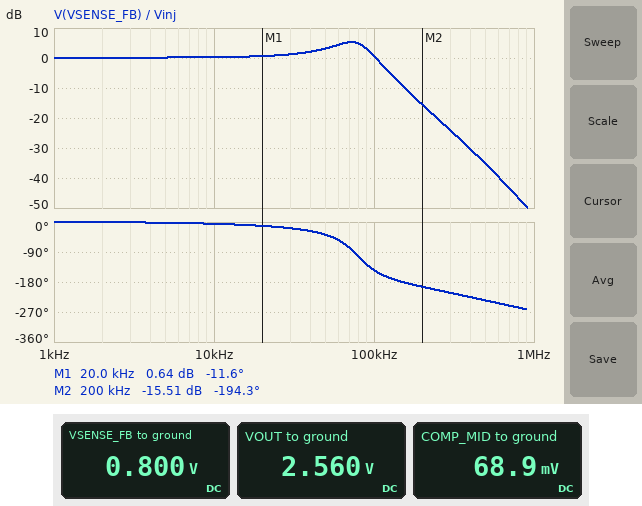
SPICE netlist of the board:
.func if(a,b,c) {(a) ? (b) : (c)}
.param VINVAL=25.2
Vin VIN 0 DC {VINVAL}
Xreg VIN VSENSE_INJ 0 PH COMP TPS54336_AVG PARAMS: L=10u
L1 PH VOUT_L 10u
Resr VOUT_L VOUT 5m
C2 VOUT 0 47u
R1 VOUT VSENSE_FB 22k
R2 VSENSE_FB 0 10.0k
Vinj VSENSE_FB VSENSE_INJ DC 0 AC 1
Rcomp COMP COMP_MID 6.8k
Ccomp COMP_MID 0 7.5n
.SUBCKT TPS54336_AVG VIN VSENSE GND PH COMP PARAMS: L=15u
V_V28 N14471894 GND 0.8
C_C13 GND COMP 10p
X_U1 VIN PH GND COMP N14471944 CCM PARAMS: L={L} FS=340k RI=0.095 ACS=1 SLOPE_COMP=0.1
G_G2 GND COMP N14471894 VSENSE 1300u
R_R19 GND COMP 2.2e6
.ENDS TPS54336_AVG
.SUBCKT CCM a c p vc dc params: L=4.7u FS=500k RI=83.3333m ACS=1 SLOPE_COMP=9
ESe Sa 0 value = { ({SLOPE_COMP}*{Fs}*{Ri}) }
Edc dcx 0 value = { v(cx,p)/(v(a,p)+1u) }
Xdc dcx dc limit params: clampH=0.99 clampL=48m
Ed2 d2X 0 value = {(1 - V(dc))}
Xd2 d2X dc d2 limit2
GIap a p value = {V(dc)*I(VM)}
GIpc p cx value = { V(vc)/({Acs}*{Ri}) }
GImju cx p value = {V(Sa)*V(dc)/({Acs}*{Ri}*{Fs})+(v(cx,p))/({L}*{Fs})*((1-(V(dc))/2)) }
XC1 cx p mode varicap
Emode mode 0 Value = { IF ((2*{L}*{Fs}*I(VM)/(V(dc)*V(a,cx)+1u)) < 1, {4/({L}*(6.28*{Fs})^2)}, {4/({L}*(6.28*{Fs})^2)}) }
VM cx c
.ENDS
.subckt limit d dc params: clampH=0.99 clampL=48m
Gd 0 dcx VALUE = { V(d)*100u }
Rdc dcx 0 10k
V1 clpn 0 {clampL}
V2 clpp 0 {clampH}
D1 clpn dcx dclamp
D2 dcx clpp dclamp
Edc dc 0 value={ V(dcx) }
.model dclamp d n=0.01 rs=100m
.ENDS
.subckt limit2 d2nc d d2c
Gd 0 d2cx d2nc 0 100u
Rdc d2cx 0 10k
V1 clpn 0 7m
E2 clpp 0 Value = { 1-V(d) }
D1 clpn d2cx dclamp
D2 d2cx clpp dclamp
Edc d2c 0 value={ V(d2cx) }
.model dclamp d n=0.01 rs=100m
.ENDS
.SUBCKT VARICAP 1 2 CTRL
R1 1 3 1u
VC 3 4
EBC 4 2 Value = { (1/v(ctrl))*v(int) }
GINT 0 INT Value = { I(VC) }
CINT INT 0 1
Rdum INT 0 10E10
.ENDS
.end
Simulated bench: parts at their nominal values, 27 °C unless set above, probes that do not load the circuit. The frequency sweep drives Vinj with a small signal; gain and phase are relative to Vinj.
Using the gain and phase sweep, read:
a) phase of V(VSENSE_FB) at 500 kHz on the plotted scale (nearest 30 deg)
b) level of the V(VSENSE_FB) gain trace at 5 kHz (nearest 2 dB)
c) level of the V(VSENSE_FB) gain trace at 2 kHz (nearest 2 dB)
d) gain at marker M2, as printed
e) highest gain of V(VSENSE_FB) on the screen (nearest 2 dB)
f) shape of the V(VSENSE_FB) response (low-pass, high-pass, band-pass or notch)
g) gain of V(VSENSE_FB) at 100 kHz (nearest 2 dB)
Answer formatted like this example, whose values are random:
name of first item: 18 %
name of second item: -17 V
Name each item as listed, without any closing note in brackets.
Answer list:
phase of V(VSENSE_FB) at 500 kHz on the plotted scale: -240 deg
level of the V(VSENSE_FB) gain trace at 5 kHz: 0 dB
level of the V(VSENSE_FB) gain trace at 2 kHz: 0 dB
gain at marker M2, as printed: -15.51 dB
highest gain of V(VSENSE_FB) on the screen: 6 dB
shape of the V(VSENSE_FB) response: low-pass
gain of V(VSENSE_FB) at 100 kHz: 0 dB
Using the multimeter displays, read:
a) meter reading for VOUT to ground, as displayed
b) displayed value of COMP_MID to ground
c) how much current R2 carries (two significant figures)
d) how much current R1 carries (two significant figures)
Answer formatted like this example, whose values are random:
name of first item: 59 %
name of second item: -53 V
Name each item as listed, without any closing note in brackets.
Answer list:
meter reading for VOUT to ground, as displayed: 2.560 V
displayed value of COMP_MID to ground: 68.9 mV
how much current R2 carries: 80 µA
how much current R1 carries: 80 µA
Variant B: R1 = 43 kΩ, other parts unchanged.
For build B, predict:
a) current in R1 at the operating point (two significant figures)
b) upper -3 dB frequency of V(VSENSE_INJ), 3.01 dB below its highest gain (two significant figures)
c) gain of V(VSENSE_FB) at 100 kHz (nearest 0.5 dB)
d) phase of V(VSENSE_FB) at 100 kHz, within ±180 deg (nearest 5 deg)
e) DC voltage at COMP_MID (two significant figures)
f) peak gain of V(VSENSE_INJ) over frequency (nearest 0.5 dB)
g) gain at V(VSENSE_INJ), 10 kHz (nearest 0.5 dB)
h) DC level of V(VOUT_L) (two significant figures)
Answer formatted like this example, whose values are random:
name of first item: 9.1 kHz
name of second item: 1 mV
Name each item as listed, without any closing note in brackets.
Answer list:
current in R1 at the operating point: 80 µA
upper -3 dB frequency of V(VSENSE_INJ), 3.01 dB below its highest gain: 150 kHz
gain of V(VSENSE_FB) at 100 kHz: -5.5 dB
phase of V(VSENSE_FB) at 100 kHz, within ±180 deg: -150 deg
DC voltage at COMP_MID: 110 mV
peak gain of V(VSENSE_INJ) over frequency: 4.5 dB
gain at V(VSENSE_INJ), 10 kHz: -15.5 dB
DC level of V(VOUT_L): 4.2 V
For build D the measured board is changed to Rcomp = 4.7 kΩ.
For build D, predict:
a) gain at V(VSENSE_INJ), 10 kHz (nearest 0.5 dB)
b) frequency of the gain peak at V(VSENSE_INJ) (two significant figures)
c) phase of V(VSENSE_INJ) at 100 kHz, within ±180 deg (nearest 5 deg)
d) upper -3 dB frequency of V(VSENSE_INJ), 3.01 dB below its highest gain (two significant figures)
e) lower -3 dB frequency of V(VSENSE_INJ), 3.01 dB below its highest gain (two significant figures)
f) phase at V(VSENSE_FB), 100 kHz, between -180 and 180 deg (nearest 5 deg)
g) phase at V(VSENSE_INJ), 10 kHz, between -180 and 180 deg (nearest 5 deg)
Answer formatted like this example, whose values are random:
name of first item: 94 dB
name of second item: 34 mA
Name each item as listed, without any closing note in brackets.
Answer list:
gain at V(VSENSE_INJ), 10 kHz: -17.0 dB
frequency of the gain peak at V(VSENSE_INJ): 71 kHz
phase of V(VSENSE_INJ) at 100 kHz, within ±180 deg: -170 deg
upper -3 dB frequency of V(VSENSE_INJ), 3.01 dB below its highest gain: 130 kHz
lower -3 dB frequency of V(VSENSE_INJ), 3.01 dB below its highest gain: 50 kHz
phase at V(VSENSE_FB), 100 kHz, between -180 and 180 deg: -155 deg
phase at V(VSENSE_INJ), 10 kHz, between -180 and 180 deg: -70 deg
